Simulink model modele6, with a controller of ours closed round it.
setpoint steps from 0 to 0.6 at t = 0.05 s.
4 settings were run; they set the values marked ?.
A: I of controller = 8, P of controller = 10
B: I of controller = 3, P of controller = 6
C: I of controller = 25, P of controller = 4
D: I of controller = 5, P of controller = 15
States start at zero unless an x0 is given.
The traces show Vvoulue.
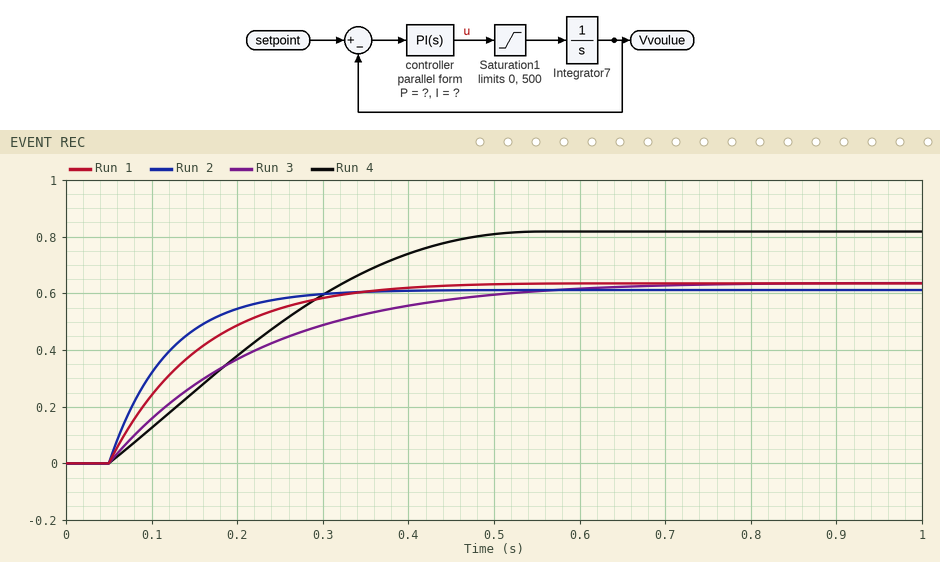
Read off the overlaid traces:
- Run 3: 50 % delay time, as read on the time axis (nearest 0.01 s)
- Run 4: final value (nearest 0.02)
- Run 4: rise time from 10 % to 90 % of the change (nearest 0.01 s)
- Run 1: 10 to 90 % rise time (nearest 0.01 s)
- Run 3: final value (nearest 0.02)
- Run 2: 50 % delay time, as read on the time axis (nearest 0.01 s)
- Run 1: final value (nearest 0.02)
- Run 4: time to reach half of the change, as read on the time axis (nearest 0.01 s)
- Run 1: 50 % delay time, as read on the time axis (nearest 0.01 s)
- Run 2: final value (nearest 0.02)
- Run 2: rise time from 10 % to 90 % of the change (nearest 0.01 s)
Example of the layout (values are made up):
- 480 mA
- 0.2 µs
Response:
- 0.17 s
- 0.82
- 0.31 s
- 0.22 s
- 0.64
- 0.10 s
- 0.64
- 0.21 s
- 0.12 s
- 0.62
- 0.15 s
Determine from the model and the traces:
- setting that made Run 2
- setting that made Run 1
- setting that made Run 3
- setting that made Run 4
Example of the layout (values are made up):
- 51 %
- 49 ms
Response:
- D
- A
- B
- C
